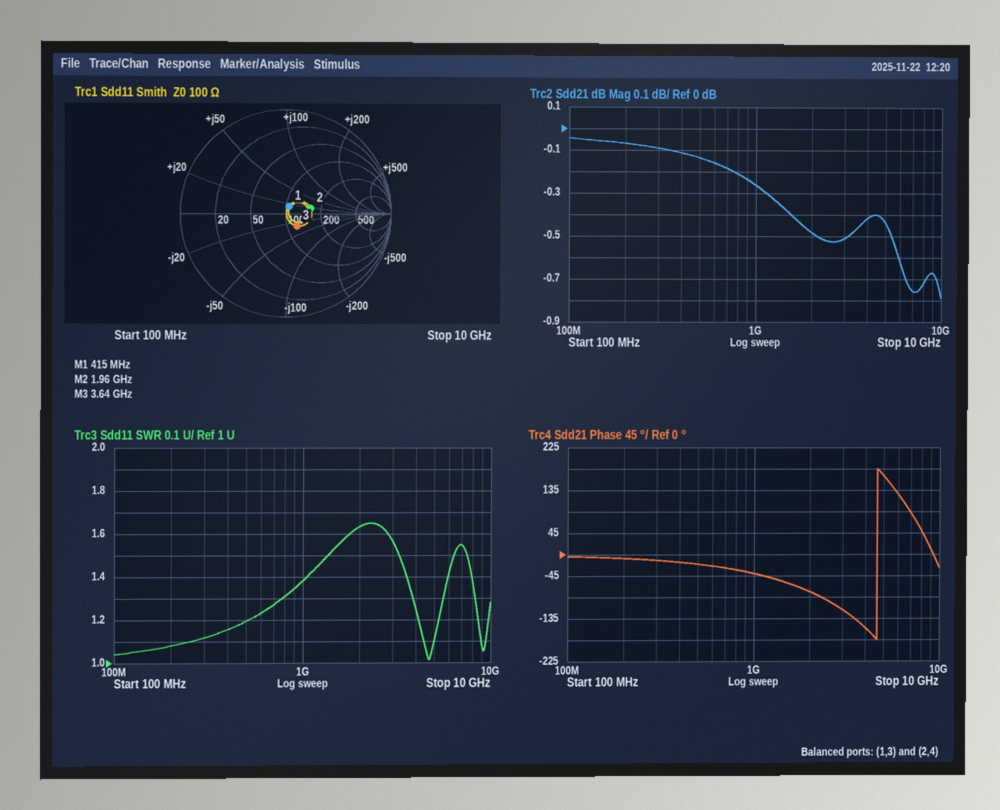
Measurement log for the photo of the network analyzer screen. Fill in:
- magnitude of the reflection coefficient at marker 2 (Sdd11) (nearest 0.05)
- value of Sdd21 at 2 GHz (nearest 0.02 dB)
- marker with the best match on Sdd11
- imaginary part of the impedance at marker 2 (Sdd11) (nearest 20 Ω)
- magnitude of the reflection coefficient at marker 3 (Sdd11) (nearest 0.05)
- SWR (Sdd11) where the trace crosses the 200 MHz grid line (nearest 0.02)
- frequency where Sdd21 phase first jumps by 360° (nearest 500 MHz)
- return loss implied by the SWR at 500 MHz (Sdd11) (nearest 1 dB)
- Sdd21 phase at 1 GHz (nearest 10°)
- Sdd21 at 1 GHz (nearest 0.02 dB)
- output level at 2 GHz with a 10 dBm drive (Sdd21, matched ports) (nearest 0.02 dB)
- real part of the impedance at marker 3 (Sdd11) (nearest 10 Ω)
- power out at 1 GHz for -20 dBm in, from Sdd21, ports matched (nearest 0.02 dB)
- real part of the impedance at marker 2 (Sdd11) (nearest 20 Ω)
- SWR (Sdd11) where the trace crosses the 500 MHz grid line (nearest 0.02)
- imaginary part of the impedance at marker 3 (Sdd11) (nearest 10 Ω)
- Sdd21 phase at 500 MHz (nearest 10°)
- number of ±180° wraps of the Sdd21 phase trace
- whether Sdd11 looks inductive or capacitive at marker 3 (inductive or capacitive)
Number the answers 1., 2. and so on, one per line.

1. 0.25
2. -0.48 dB
3. marker 1
4. +20 Ω
5. 0.15
6. 1.08
7. 4.5 GHz
8. 21 dB
9. -40°
10. -0.26 dB
11. 9.52 dBm
12. 120 Ω
13. -20.26 dBm
14. 160 Ω
15. 1.20
16. -30 Ω
17. -20°
18. 1
19. capacitive
